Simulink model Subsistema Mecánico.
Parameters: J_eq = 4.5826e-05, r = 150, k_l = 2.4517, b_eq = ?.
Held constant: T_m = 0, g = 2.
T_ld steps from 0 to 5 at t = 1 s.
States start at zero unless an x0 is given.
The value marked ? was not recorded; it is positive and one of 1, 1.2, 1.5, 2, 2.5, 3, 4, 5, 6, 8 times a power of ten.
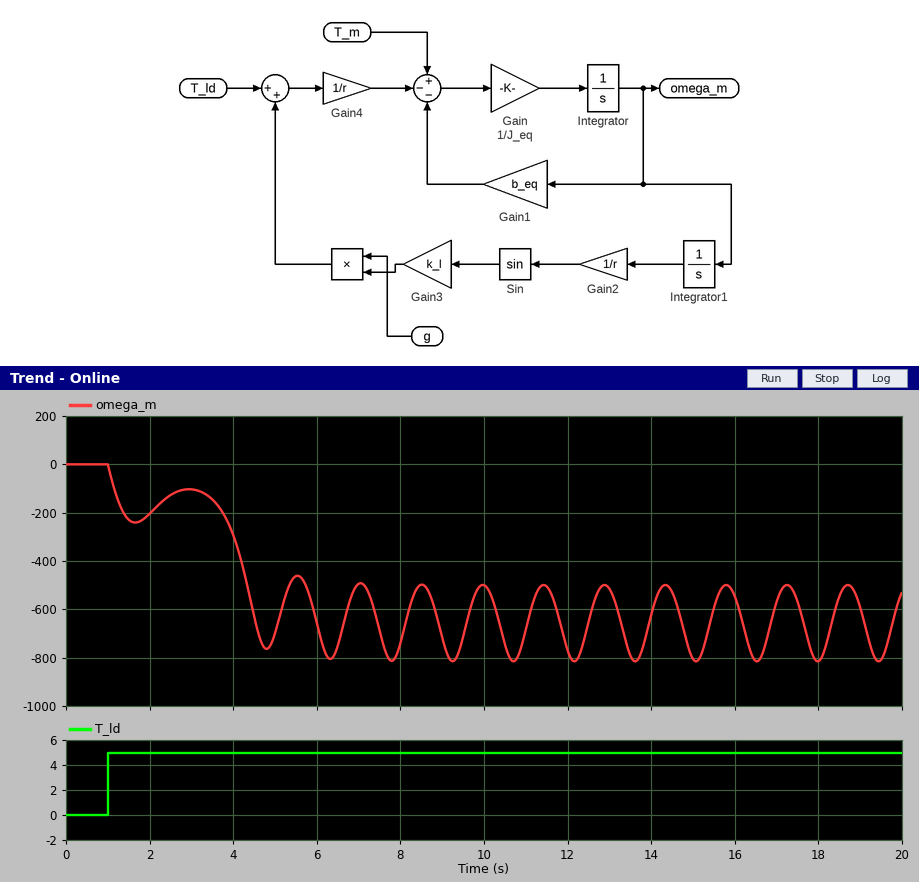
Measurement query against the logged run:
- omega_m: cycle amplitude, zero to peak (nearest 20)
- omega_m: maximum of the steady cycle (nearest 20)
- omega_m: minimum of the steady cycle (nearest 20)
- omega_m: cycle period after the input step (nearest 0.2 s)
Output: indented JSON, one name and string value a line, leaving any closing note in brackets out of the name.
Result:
{
  "omega_m: cycle amplitude, zero to peak": "160",
  "omega_m: maximum of the steady cycle": "-500",
  "omega_m: minimum of the steady cycle": "-820",
  "omega_m: cycle period after the input step": "1.4 s"
}
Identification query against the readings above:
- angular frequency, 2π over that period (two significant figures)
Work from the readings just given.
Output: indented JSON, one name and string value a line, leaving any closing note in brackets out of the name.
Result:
{
  "angular frequency, 2π over that period": "4.5 rad/s"
}
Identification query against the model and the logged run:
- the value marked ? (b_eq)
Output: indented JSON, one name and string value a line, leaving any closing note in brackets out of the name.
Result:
{
  "the value marked ?": "5e-05"
}
